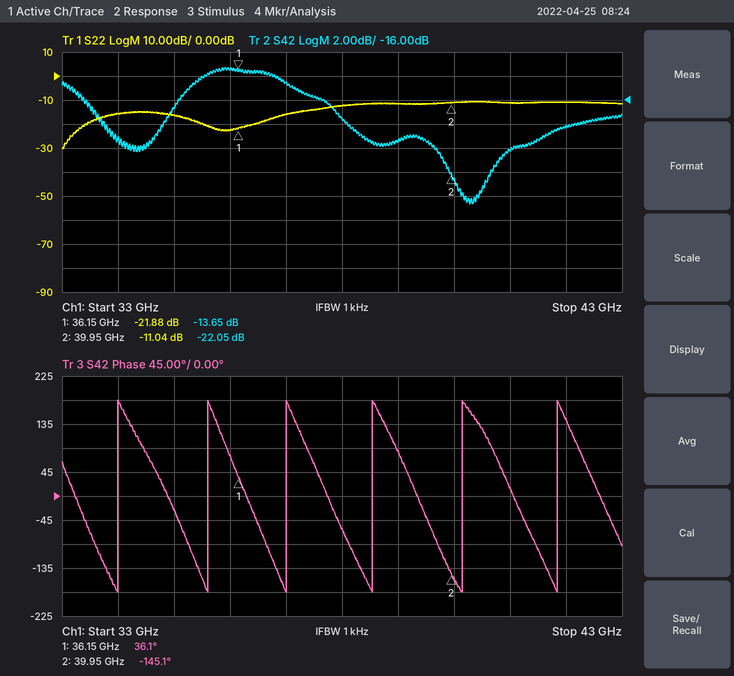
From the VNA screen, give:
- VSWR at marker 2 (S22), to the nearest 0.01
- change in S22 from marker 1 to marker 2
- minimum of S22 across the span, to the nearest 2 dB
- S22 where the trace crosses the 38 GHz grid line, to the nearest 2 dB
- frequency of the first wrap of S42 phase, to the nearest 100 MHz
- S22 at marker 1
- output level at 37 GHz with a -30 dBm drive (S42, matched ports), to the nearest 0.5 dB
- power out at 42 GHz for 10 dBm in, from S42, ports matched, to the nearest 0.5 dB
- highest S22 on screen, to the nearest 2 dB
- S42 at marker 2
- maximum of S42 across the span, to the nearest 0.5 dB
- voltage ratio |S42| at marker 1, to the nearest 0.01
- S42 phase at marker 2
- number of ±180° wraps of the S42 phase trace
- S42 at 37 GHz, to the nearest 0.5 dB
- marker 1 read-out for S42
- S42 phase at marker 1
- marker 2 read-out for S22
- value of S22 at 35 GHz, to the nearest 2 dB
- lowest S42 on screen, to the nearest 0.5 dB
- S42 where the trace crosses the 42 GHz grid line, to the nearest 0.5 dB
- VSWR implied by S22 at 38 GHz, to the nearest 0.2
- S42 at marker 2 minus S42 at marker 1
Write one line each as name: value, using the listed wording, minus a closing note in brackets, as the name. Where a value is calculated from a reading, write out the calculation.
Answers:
VSWR at marker 2 (S22), to the nearest 0.01: (1 + 0.2805)/(1 − 0.2805) ≈ 1.78
change in S22 from marker 1 to marker 2: -11.04 − (-21.88) = 10.84 dB
minimum of S22 across the span, to the nearest 2 dB: -30 dB
S22 where the trace crosses the 38 GHz grid line, to the nearest 2 dB: -12 dB
frequency of the first wrap of S42 phase, to the nearest 100 MHz: 34.0 GHz
S22 at marker 1: -21.88 dB
output level at 37 GHz with a -30 dBm drive (S42, matched ports), to the nearest 0.5 dB: -30 dBm + (-14.5 dB) = -44.5 dBm
power out at 42 GHz for 10 dBm in, from S42, ports matched, to the nearest 0.5 dB: 10 dBm + (-18.0 dB) = -8.0 dBm
highest S22 on screen, to the nearest 2 dB: -10 dB
S42 at marker 2: -22.05 dB
maximum of S42 across the span, to the nearest 0.5 dB: -13.5 dB
voltage ratio |S42| at marker 1, to the nearest 0.01: 10^(-13.65/20) ≈ 0.21
S42 phase at marker 2: -145.1°
number of ±180° wraps of the S42 phase trace: 6
S42 at 37 GHz, to the nearest 0.5 dB: -14.5 dB
marker 1 read-out for S42: -13.65 dB
S42 phase at marker 1: 36.1°
marker 2 read-out for S22: -11.04 dB
value of S22 at 35 GHz, to the nearest 2 dB: -16 dB
lowest S42 on screen, to the nearest 0.5 dB: -24.5 dB
S42 where the trace crosses the 42 GHz grid line, to the nearest 0.5 dB: -18.0 dB
VSWR implied by S22 at 38 GHz, to the nearest 0.2: |Γ| = 10^(-12/20) = 0.2512; VSWR = (1 + 0.2512)/(1 − 0.2512) ≈ 1.67, so 1.6 to the nearest 0.2
S42 at marker 2 minus S42 at marker 1: -22.05 − (-13.65) = -8.40 dB
